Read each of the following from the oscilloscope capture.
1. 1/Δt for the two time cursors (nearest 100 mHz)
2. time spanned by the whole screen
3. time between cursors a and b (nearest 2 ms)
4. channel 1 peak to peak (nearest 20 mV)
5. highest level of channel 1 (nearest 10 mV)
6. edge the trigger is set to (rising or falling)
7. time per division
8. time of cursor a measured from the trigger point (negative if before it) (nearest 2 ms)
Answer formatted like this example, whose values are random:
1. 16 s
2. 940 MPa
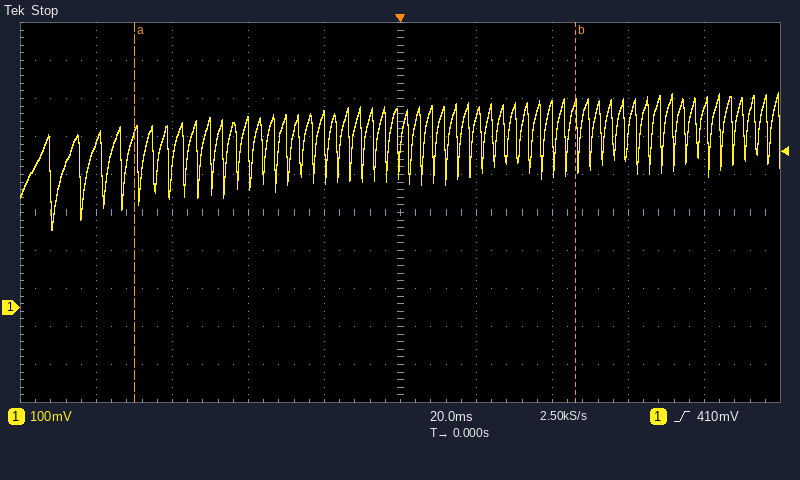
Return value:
1. 8.6 Hz
2. 200 ms
3. 116 ms
4. 360 mV
5. 570 mV
6. rising
7. 20 ms
8. -70 ms
